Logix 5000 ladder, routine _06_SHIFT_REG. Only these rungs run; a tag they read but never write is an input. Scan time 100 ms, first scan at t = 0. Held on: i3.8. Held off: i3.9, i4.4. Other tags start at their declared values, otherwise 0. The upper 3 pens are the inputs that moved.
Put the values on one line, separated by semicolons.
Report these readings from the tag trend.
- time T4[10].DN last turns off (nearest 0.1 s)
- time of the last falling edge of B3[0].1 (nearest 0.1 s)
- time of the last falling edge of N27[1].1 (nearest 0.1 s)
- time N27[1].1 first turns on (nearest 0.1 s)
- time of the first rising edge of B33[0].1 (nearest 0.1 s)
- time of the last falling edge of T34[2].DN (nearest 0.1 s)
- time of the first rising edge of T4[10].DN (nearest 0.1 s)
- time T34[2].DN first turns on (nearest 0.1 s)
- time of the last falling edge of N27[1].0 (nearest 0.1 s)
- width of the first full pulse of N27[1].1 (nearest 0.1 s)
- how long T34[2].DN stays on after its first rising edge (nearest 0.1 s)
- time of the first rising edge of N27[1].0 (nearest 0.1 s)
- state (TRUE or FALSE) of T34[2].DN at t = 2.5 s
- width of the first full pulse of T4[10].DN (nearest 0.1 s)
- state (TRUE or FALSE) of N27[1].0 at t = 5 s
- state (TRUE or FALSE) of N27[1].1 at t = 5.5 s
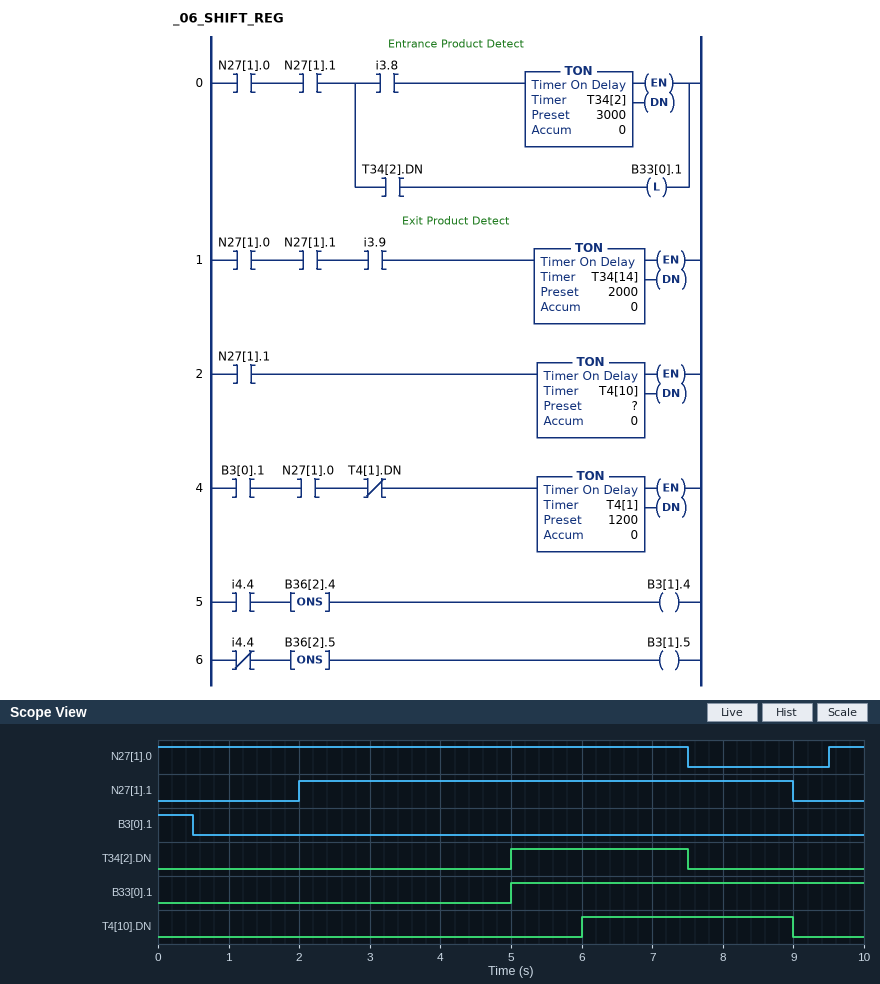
9.0 s; 0.5 s; 9.0 s; 2.0 s; 5.0 s; 7.5 s; 6.0 s; 5.0 s; 7.5 s; 7.0 s; 2.5 s; 9.5 s; FALSE; 3.0 s; TRUE; TRUE
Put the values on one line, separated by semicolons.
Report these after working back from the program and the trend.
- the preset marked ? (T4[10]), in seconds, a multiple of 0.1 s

4.0 s
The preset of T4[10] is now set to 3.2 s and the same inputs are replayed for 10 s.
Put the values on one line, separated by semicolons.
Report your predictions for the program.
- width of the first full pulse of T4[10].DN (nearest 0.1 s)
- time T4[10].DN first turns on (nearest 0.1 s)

3.8 s; 5.2 s
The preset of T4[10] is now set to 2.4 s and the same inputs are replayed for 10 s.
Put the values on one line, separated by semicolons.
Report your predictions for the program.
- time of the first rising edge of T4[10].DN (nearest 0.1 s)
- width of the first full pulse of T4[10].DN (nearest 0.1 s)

4.4 s; 4.6 s
